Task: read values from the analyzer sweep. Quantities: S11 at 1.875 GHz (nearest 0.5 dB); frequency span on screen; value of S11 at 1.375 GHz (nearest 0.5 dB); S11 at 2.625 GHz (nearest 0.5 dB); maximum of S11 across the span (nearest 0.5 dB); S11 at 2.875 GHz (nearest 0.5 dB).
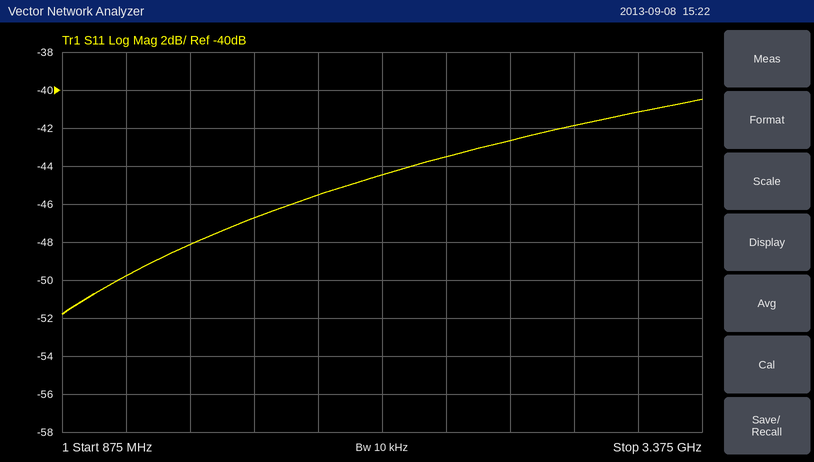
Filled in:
-45.5 dB
2.5 GHz
-48.0 dB
-42.5 dB
-40.5 dB
-42.0 dB
